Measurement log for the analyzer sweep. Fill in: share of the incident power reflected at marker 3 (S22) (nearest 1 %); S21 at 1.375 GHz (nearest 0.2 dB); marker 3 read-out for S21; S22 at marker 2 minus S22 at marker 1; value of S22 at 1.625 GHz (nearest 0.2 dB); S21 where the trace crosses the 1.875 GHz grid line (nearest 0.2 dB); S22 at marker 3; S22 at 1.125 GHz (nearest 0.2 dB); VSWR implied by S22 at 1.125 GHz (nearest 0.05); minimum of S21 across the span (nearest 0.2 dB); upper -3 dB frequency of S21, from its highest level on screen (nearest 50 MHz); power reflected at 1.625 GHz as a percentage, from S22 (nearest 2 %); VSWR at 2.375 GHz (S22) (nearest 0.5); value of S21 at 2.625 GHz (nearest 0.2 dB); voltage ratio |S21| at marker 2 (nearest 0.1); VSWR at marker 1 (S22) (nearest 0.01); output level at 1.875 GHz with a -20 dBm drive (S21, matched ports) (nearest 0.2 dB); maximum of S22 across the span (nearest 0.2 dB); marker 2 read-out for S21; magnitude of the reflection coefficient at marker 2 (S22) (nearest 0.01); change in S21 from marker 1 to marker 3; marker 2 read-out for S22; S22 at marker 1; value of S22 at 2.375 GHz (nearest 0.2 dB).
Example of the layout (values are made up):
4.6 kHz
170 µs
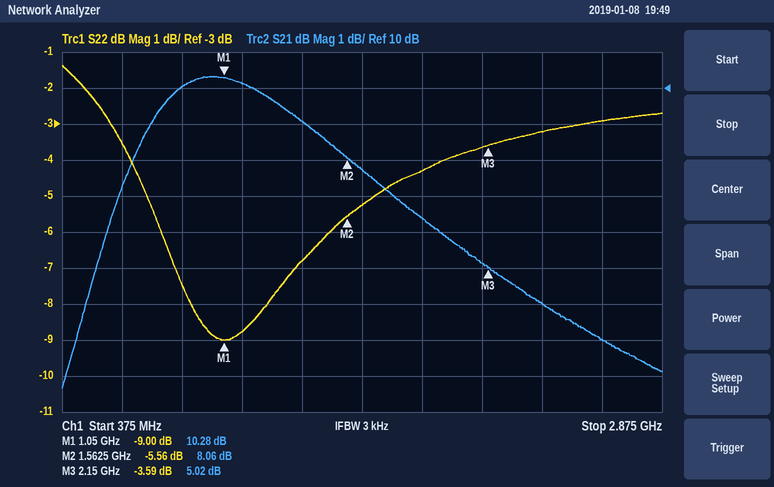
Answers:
44 %
9.0 dB
5.02 dB
3.44 dB
-5.2 dB
6.4 dB
-3.59 dB
-8.8 dB
2.15
1.6 dB
1.70 GHz
30 %
5.5
3.0 dB
2.5
2.10
-13.6 dBm
-1.4 dB
8.06 dB
0.53
-5.26 dB
-5.56 dB
-9.00 dB
-3.2 dB
